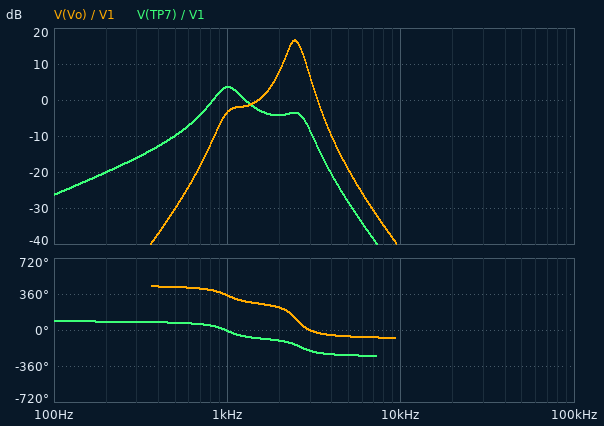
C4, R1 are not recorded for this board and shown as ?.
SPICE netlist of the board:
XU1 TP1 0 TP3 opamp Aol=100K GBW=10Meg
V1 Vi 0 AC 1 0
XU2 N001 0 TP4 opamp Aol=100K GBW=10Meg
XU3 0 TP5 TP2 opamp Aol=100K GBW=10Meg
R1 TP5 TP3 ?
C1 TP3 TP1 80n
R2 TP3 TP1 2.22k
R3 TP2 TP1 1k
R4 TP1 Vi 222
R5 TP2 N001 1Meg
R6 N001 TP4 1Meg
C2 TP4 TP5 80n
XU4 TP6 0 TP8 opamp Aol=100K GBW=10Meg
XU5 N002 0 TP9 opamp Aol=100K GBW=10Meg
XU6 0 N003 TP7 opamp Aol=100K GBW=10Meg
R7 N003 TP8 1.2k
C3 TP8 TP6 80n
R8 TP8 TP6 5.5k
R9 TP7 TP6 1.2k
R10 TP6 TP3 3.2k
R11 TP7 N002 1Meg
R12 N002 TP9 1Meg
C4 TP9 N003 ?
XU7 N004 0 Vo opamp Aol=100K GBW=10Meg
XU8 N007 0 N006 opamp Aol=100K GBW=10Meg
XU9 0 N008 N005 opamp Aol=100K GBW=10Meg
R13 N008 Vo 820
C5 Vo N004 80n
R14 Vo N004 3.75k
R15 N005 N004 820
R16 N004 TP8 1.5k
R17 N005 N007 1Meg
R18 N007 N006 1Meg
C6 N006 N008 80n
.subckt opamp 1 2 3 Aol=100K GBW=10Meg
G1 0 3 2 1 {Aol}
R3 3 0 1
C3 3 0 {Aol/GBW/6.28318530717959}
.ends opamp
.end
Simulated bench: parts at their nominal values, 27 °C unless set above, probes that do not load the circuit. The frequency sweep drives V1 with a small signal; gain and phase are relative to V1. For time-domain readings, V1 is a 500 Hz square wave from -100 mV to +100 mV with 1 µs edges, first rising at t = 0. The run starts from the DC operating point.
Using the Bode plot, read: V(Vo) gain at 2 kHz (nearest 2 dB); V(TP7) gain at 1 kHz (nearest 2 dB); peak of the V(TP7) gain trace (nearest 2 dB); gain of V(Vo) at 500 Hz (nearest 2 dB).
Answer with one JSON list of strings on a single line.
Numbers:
["8 dB", "4 dB", "4 dB", "-30 dB"]
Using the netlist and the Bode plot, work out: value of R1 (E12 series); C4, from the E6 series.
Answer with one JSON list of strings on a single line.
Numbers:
["560 Ω", "220 nF"]
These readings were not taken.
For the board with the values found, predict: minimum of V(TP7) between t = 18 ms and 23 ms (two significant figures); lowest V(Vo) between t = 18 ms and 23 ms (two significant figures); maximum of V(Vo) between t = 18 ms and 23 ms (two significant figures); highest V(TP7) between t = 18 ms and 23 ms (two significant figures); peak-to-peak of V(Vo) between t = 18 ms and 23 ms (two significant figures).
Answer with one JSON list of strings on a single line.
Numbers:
["-82 mV", "-220 mV", "220 mV", "82 mV", "440 mV"]
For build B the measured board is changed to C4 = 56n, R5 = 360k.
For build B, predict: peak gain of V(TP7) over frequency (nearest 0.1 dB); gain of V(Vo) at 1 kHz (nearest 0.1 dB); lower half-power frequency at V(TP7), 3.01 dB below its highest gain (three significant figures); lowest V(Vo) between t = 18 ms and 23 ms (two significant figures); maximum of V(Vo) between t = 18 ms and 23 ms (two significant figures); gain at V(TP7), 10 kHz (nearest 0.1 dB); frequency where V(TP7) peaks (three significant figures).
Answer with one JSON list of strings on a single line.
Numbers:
["24.5 dB", "-10.9 dB", "1.70 kHz", "-300 mV", "300 mV", "-37.1 dB", "1.93 kHz"]
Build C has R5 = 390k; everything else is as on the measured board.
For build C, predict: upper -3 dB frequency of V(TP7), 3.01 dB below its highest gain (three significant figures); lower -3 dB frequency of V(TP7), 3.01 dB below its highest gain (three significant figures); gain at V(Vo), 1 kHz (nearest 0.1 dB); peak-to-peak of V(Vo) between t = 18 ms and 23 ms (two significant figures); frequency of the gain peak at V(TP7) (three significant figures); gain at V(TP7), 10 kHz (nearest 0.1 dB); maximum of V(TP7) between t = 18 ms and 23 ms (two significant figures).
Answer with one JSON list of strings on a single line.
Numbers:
["1.29 kHz", "864 Hz", "6.5 dB", "490 mV", "1.02 kHz", "-49.2 dB", "190 mV"]
